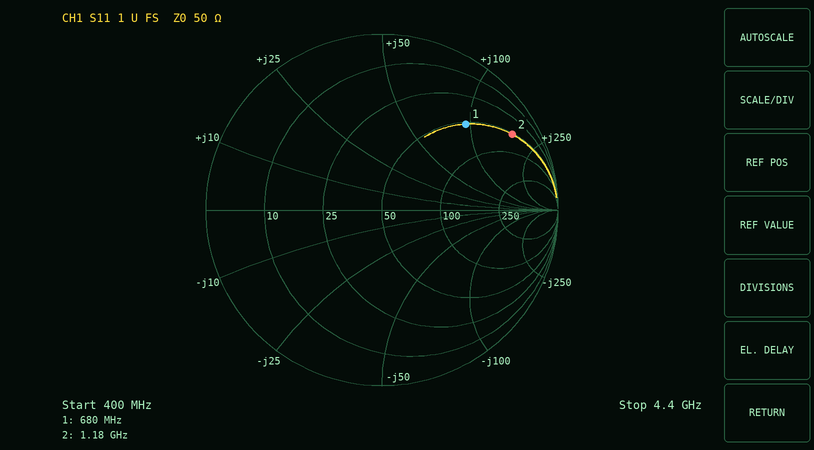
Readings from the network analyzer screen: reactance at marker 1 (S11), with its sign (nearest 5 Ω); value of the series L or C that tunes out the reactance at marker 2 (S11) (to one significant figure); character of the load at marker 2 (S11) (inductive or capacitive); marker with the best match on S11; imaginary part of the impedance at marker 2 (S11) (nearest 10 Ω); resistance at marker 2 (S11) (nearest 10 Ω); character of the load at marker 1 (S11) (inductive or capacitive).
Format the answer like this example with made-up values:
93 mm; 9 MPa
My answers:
+95 Ω; 800 fF; inductive; marker 1; +170 Ω; 50 Ω; inductive
